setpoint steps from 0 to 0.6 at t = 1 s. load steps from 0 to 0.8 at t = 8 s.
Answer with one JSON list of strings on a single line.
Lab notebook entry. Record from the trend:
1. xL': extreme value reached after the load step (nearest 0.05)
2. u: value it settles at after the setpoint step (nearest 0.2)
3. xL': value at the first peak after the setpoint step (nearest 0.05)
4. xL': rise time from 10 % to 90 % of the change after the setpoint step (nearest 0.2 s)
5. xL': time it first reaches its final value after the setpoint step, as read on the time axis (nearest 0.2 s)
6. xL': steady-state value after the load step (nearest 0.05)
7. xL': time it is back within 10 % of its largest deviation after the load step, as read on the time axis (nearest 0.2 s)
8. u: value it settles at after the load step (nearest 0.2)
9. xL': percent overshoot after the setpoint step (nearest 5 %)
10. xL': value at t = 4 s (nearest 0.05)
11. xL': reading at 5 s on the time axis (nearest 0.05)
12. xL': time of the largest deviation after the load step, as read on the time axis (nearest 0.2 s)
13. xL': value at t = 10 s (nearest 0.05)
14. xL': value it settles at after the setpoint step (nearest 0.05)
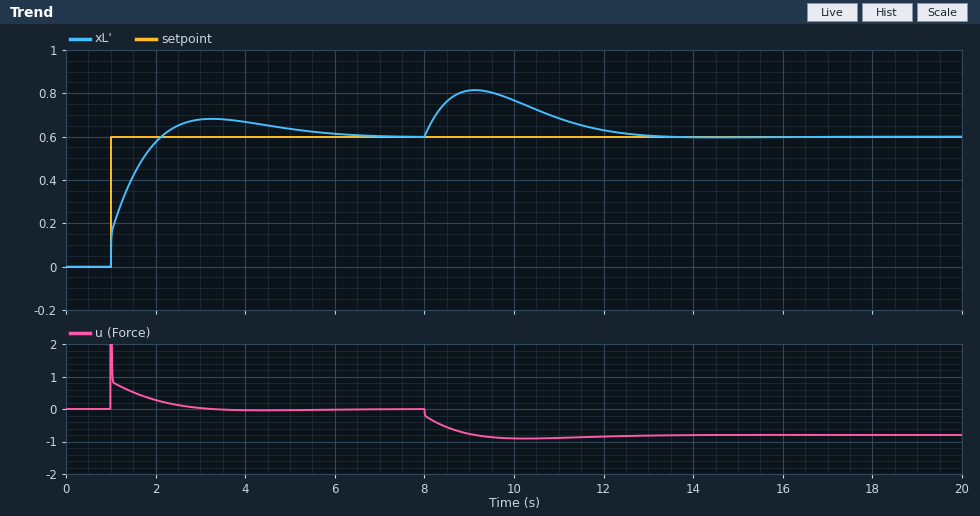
["0.80", "0.0", "0.70", "0.8 s", "2.2 s", "0.60", "12.2 s", "-0.8", "15 %", "0.65", "0.65", "9.2 s", "0.75", "0.60"]
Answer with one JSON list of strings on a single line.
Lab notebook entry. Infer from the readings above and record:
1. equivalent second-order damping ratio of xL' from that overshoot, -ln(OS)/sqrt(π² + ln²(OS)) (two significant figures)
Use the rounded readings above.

["0.52"]
